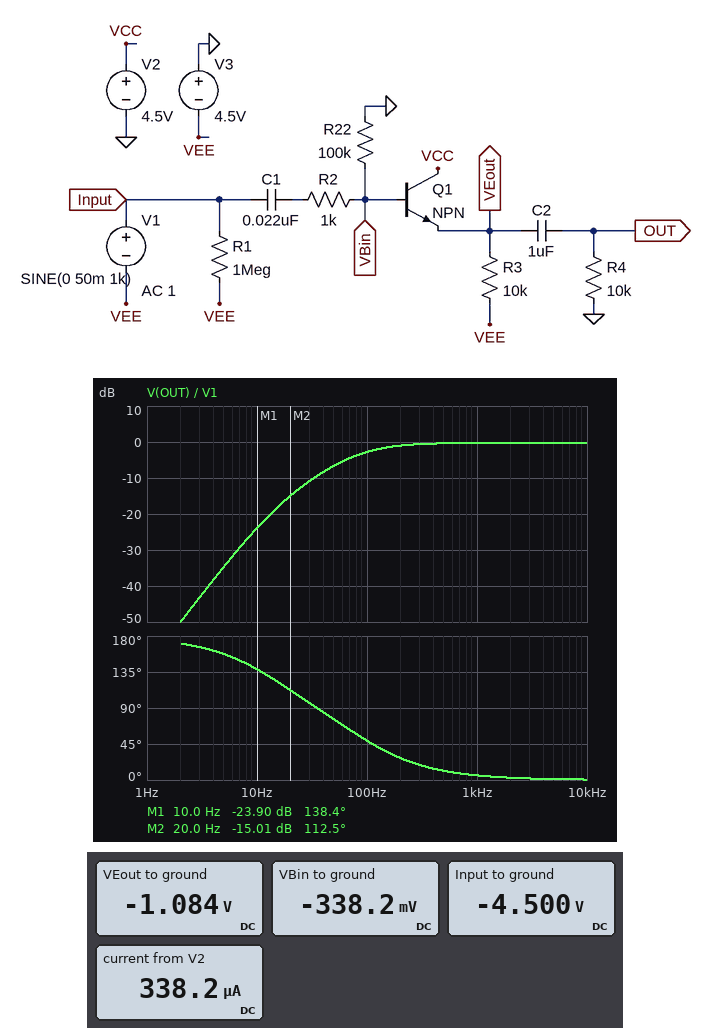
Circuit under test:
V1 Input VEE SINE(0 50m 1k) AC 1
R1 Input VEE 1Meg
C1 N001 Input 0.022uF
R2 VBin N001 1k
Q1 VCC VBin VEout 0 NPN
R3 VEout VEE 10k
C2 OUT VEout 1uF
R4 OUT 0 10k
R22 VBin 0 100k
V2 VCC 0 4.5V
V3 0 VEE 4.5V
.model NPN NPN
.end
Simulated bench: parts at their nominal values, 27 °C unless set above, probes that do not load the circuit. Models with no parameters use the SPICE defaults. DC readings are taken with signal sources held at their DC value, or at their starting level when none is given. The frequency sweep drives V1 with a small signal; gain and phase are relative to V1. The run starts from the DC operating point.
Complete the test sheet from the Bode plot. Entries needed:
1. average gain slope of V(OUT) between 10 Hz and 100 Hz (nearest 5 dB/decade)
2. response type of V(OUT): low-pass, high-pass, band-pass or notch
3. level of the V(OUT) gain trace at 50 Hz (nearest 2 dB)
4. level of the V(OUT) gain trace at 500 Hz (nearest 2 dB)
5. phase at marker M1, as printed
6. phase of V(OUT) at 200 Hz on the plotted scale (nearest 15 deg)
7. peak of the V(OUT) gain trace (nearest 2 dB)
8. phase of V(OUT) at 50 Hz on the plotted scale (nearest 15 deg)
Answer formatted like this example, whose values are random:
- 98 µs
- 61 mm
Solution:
- 20 dB/decade
- high-pass
- -6 dB
- 0 dB
- 138.4 deg
- 30 deg
- 0 dB
- 75 deg
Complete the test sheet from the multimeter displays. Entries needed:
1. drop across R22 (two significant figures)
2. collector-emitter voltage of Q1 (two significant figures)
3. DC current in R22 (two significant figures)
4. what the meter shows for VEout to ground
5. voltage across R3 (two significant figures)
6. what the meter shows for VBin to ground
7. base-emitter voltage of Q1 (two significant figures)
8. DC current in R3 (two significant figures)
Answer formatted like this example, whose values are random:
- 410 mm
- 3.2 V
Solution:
- 340 mV
- 5.6 V
- 3.4 µA
- -1.084 V
- 3.4 V
- -338.2 mV
- 750 mV
- 340 µA
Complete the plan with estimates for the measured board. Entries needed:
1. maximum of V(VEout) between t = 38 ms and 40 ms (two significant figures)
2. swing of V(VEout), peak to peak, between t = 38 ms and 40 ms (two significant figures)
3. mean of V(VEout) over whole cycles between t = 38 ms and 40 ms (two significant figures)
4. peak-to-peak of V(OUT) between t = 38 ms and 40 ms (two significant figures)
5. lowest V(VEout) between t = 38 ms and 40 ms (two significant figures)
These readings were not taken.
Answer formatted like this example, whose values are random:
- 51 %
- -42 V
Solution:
- -1.0 V
- 97 mV
- -1.1 V
- 97 mV
- -1.1 V
